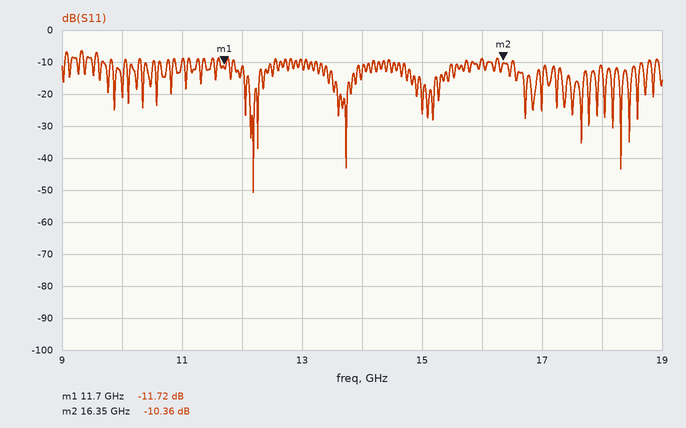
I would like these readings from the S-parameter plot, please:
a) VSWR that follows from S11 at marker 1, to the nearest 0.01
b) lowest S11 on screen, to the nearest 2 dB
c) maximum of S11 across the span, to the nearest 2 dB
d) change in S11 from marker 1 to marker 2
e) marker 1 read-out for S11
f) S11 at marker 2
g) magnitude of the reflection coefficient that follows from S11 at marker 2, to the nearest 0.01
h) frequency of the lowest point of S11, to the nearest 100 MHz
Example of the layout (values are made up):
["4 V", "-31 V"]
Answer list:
["1.70", "-50 dB", "-6 dB", "1.36 dB", "-11.72 dB", "-10.36 dB", "0.30", "12.2 GHz"]
